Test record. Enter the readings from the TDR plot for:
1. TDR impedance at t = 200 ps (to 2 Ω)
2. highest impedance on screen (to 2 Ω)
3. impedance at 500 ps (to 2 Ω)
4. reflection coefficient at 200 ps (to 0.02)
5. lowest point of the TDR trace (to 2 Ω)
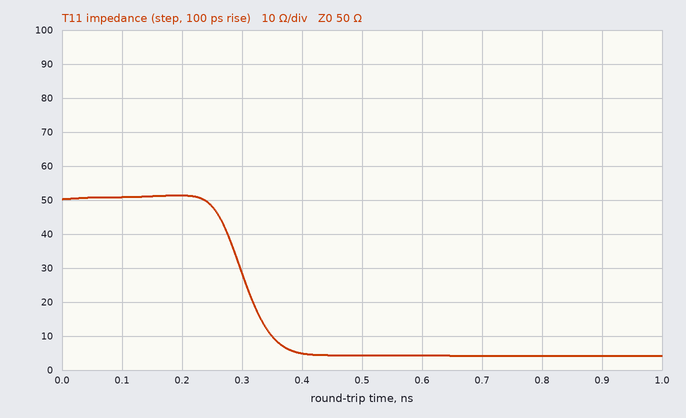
52 Ω
52 Ω
4 Ω
+0.02
4 Ω
